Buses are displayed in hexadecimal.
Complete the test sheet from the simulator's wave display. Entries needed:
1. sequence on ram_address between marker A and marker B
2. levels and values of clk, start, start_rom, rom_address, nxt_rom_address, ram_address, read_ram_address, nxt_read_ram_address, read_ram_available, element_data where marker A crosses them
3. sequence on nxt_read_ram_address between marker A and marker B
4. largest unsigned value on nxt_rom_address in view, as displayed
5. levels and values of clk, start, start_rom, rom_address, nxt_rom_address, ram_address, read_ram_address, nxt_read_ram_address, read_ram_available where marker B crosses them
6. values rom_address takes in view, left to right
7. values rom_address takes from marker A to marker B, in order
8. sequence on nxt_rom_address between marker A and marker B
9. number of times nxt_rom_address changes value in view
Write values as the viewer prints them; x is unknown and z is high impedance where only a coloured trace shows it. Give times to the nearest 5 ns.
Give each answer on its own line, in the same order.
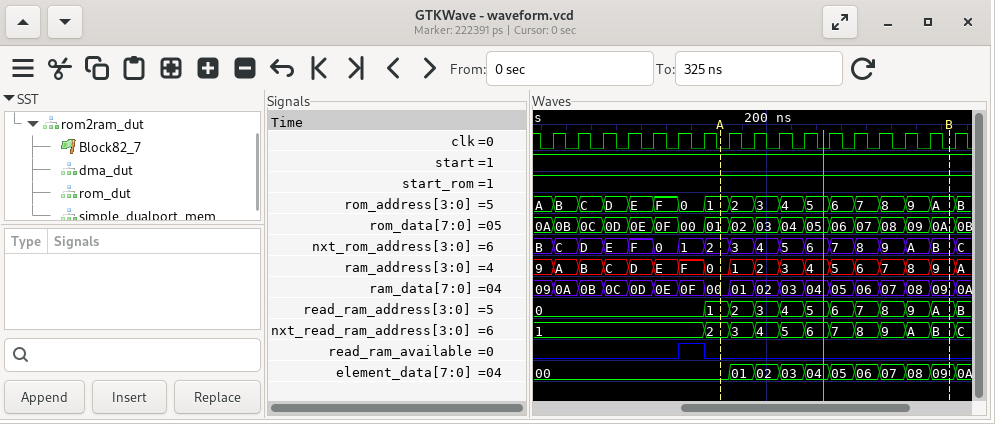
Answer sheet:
0, 1, 2, 3, 4, 5, 6, 7, 8, 9
clk=0, start=1, start_rom=1, rom_address=1, nxt_rom_address=2, ram_address=0, read_ram_address=1, nxt_read_ram_address=2, read_ram_available=0, element_data=00
2, 3, 4, 5, 6, 7, 8, 9, A, B
F
clk=0, start=1, start_rom=1, rom_address=A, nxt_rom_address=B, ram_address=9, read_ram_address=A, nxt_read_ram_address=B, read_ram_available=0
A, B, C, D, E, F, 0, 1, 2, 3, 4, 5, 6, 7, 8, 9, A, B
1, 2, 3, 4, 5, 6, 7, 8, 9, A
2, 3, 4, 5, 6, 7, 8, 9, A, B
17
